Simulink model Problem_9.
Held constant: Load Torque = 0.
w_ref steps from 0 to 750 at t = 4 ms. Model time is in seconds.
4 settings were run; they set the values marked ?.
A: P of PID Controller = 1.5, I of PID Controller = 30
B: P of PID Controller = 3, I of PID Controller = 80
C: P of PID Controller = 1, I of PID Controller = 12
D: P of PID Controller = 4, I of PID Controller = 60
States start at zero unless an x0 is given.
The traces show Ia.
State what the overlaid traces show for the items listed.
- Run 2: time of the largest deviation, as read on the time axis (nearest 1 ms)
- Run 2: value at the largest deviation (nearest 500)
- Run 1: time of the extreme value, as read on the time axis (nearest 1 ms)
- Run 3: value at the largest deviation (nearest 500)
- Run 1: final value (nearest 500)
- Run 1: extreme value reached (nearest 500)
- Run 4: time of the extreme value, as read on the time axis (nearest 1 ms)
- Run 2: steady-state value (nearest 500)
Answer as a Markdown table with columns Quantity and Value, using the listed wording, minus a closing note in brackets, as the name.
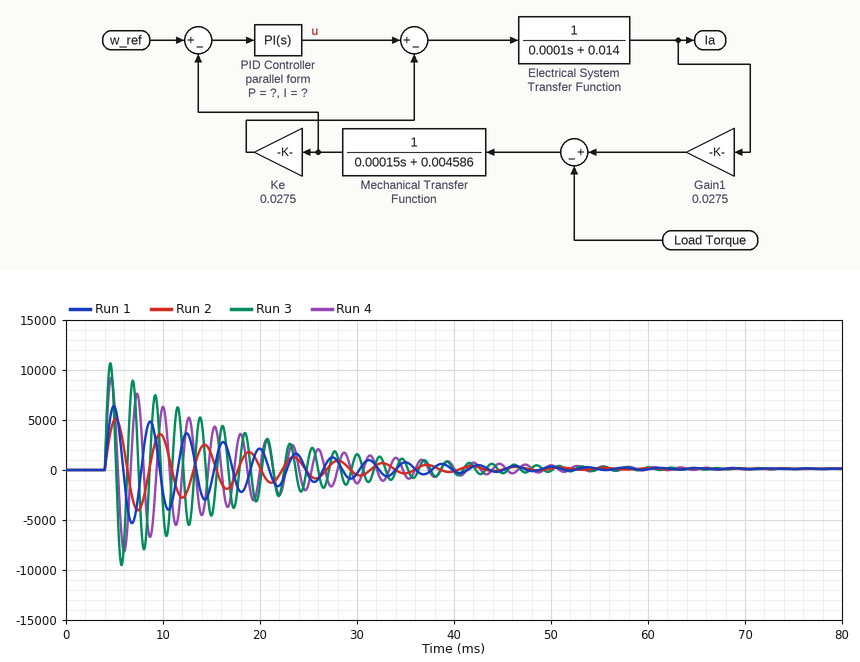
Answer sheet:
| Quantity | Value |
|---|---|
| Run 2: time of the largest deviation, as read on the time axis | 5 ms |
| Run 2: value at the largest deviation | 5000 |
| Run 1: time of the extreme value, as read on the time axis | 5 ms |
| Run 3: value at the largest deviation | 10500 |
| Run 1: final value | 0 |
| Run 1: extreme value reached | 6500 |
| Run 4: time of the extreme value, as read on the time axis | 5 ms |
| Run 2: steady-state value | 0 |
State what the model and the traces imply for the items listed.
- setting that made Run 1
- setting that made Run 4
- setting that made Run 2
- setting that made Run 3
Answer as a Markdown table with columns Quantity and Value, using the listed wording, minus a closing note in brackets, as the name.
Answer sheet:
| Quantity | Value |
|---|---|
| setting that made Run 1 | A |
| setting that made Run 4 | B |
| setting that made Run 2 | C |
| setting that made Run 3 | D |
